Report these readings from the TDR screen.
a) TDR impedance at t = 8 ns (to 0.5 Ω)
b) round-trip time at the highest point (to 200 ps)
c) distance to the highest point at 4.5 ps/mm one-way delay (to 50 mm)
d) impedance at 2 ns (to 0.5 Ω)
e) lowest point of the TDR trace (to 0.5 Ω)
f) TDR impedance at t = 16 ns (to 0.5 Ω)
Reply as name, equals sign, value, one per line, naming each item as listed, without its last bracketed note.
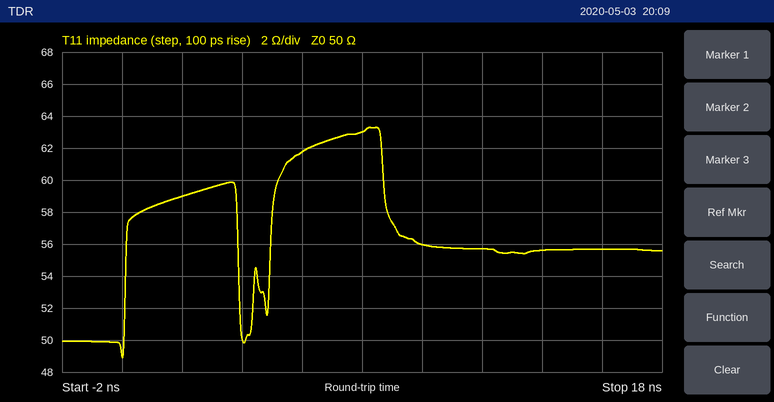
TDR impedance at t = 8 ns = 63.0 Ω
round-trip time at the highest point = 8.4 ns
distance to the highest point at 4.5 ps/mm one-way delay = 950 mm
impedance at 2 ns = 59.0 Ω
lowest point of the TDR trace = 49.0 Ω
TDR impedance at t = 16 ns = 55.5 Ω
